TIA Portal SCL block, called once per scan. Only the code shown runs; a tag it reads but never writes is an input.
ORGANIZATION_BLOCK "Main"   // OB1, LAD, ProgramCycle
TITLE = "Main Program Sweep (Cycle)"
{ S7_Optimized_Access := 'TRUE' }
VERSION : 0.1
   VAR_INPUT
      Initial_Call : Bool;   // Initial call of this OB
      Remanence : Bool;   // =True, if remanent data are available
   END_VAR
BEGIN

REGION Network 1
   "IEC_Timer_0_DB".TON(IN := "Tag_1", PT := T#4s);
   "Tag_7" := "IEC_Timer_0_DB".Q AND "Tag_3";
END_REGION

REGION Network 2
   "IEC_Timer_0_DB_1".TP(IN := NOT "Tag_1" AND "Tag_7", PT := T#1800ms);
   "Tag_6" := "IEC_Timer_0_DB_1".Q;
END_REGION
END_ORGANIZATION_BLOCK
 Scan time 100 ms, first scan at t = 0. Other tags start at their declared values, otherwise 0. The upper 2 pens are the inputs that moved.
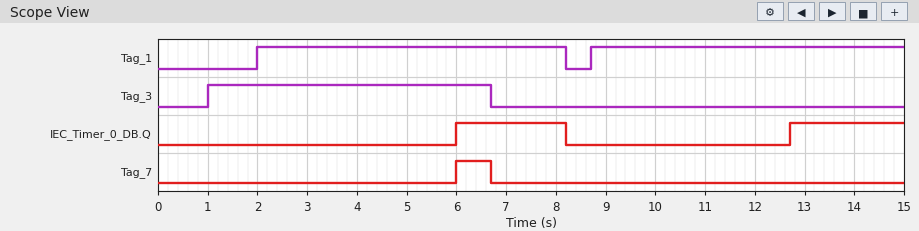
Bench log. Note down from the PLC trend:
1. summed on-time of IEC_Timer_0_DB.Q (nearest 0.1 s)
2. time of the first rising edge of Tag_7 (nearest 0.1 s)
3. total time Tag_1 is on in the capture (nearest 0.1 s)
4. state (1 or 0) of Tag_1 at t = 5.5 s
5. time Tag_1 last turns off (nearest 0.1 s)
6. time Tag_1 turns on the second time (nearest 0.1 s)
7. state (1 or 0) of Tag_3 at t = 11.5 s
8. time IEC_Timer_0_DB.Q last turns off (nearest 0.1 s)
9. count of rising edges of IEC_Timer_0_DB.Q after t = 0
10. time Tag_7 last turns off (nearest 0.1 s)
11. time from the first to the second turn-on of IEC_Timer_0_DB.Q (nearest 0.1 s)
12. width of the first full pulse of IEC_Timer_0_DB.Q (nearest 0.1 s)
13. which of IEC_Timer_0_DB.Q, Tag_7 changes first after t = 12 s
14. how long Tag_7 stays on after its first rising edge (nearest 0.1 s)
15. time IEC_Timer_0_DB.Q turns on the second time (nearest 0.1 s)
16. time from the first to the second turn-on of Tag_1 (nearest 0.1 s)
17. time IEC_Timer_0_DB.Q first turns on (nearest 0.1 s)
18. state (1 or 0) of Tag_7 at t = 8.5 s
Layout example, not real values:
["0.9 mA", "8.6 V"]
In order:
["4.5 s", "6.0 s", "12.5 s", "1", "8.2 s", "8.7 s", "0", "8.2 s", "2", "6.7 s", "6.7 s", "2.2 s", "IEC_Timer_0_DB.Q", "0.7 s", "12.7 s", "6.7 s", "6.0 s", "0"]
